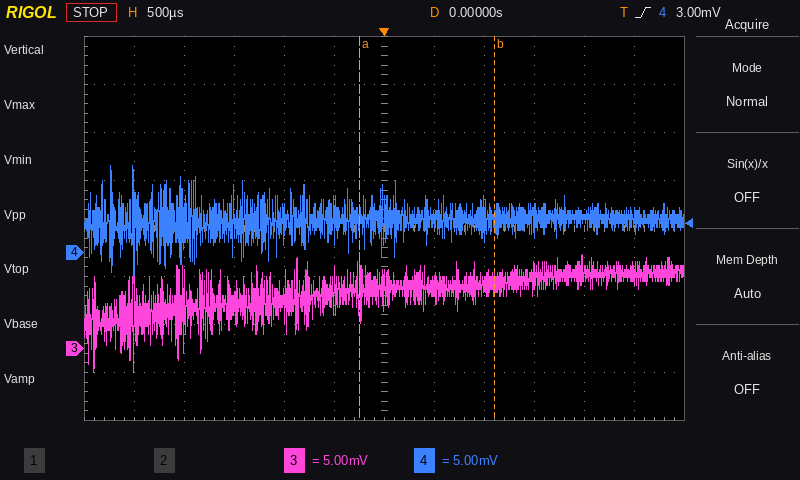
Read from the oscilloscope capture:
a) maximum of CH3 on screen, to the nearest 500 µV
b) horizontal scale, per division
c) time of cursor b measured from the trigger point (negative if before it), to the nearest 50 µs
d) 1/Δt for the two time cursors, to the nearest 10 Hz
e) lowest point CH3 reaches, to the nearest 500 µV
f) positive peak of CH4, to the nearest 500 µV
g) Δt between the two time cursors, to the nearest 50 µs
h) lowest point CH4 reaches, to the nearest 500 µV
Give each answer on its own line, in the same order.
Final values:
10.0 mV
500 µs
+1.10 ms
740 Hz
-2.5 mV
9.0 mV
1.35 ms
-3.0 mV
